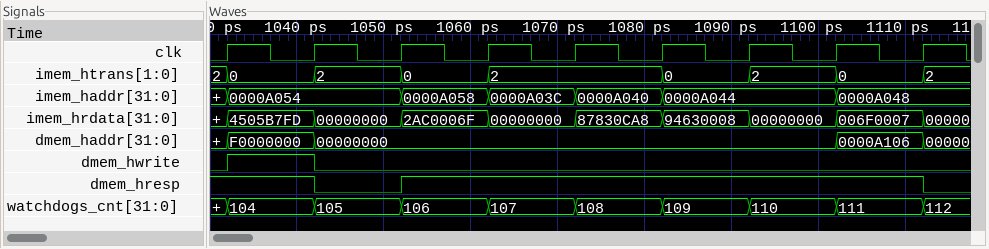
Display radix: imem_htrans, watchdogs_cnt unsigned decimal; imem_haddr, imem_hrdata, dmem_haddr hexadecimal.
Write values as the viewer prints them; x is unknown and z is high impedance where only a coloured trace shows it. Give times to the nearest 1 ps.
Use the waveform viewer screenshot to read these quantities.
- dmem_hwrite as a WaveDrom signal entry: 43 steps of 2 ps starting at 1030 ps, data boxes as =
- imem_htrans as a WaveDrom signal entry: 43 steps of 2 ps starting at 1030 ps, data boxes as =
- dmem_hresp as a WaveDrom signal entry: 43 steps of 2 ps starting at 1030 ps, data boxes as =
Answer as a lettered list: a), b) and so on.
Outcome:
a) {name: 'dmem_hwrite', wave: '01....0....................................'}
b) {name: 'imem_htrans', wave: '==....=....=....=.........=....=....=....=.', data: '2 0 2 0 2 0 2 0 2'}
c) {name: 'dmem_hresp', wave: '1.....0....1.............................0.'}
